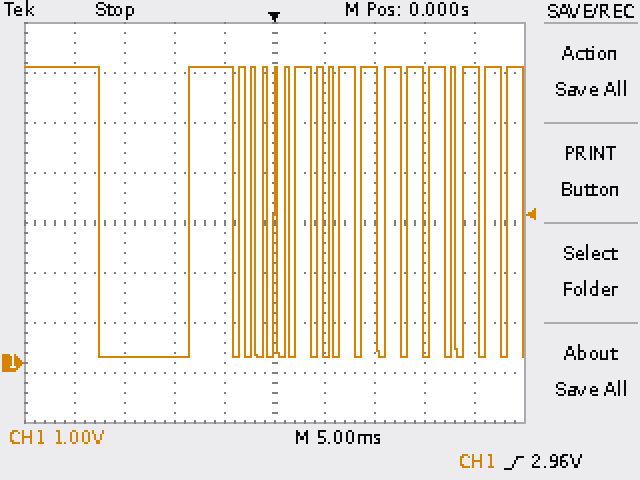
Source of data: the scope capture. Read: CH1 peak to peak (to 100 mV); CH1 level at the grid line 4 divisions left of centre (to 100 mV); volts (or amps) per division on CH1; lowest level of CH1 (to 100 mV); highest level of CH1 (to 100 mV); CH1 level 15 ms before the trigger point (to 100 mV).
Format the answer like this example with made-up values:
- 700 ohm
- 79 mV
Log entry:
- 5.8 V
- 5.9 V
- 1 V
- 100 mV
- 5.9 V
- 100 mV
